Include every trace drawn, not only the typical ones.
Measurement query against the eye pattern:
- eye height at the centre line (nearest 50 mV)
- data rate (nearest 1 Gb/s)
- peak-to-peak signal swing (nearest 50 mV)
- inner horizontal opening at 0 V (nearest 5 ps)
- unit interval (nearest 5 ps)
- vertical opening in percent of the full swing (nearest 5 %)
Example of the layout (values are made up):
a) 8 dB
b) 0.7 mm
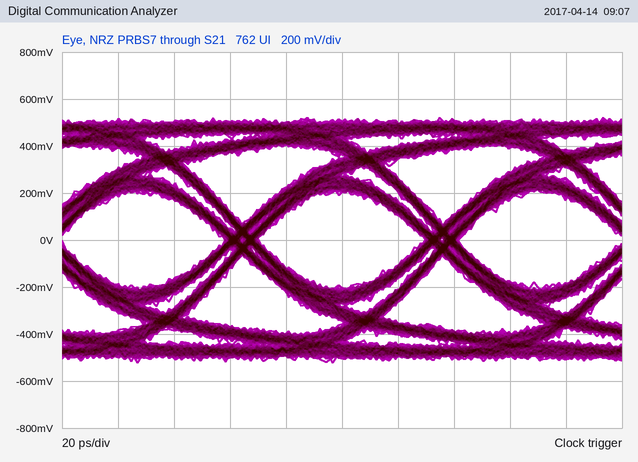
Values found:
a) 400 mV
b) 14 Gb/s
c) 1.05 V
d) 60 ps
e) 70 ps
f) 40 %
